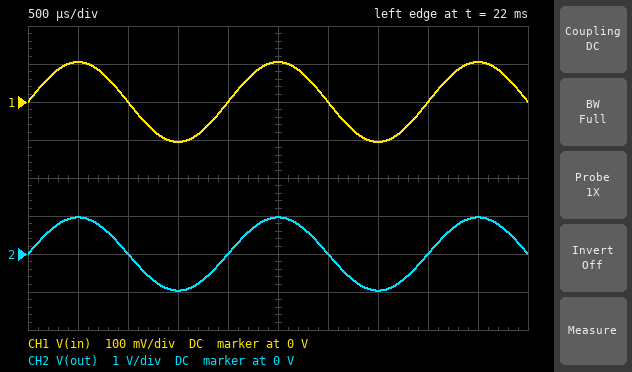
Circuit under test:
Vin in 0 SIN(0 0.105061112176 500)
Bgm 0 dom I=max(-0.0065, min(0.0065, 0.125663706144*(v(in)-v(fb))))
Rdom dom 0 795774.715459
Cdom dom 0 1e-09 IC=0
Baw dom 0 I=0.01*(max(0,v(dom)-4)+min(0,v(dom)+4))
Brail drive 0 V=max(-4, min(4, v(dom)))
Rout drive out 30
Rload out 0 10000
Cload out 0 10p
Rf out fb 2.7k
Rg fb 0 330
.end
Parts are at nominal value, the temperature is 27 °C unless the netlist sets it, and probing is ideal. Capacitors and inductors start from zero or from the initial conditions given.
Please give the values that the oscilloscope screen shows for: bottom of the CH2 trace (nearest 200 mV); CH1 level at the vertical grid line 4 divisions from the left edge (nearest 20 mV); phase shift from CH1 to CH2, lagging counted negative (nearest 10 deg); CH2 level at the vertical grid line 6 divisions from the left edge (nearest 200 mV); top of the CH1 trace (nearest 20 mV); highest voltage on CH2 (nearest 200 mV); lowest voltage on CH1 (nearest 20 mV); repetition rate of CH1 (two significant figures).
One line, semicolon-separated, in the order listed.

-1.0 V; 0 V; 0 deg; 0 V; 100 mV; 1.0 V; -100 mV; 500 Hz
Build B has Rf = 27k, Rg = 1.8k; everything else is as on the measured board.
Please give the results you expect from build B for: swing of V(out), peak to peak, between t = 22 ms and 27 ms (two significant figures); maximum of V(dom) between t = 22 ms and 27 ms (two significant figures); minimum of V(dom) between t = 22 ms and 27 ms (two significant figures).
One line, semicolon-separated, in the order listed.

3.4 V; 1.7 V; -1.7 V
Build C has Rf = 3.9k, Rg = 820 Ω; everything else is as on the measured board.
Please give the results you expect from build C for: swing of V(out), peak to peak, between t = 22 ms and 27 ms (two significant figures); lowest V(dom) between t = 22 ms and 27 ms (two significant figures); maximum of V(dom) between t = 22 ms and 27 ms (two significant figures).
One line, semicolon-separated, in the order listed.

1.2 V; -610 mV; 610 mV
